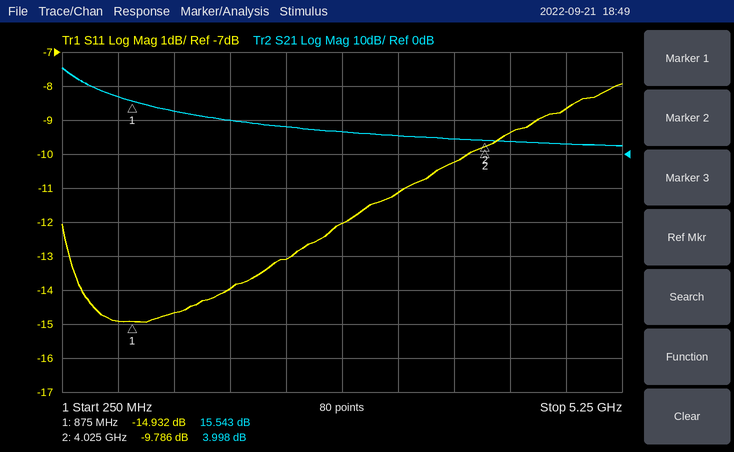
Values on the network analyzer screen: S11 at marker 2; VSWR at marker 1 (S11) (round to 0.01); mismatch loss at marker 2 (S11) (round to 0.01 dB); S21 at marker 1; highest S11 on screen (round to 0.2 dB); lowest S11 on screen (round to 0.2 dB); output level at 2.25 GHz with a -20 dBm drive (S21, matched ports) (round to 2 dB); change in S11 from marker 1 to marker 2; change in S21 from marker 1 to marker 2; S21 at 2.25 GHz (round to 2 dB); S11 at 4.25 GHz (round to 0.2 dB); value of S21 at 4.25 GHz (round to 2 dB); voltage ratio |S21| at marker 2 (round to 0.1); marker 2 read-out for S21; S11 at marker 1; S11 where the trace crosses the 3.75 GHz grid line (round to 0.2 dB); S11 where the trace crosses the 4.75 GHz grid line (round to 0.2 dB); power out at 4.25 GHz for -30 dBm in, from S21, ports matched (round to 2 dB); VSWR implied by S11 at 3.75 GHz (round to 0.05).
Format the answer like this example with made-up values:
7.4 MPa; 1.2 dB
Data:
-9.786 dB; 1.44; 0.48 dB; 15.543 dB; -8.0 dB; -15.0 dB; -12 dBm; 5.146 dB; -11.545 dB; 8 dB; -9.4 dB; 4 dB; 1.6; 3.998 dB; -14.932 dB; -10.2 dB; -8.6 dB; -26 dBm; 1.90
